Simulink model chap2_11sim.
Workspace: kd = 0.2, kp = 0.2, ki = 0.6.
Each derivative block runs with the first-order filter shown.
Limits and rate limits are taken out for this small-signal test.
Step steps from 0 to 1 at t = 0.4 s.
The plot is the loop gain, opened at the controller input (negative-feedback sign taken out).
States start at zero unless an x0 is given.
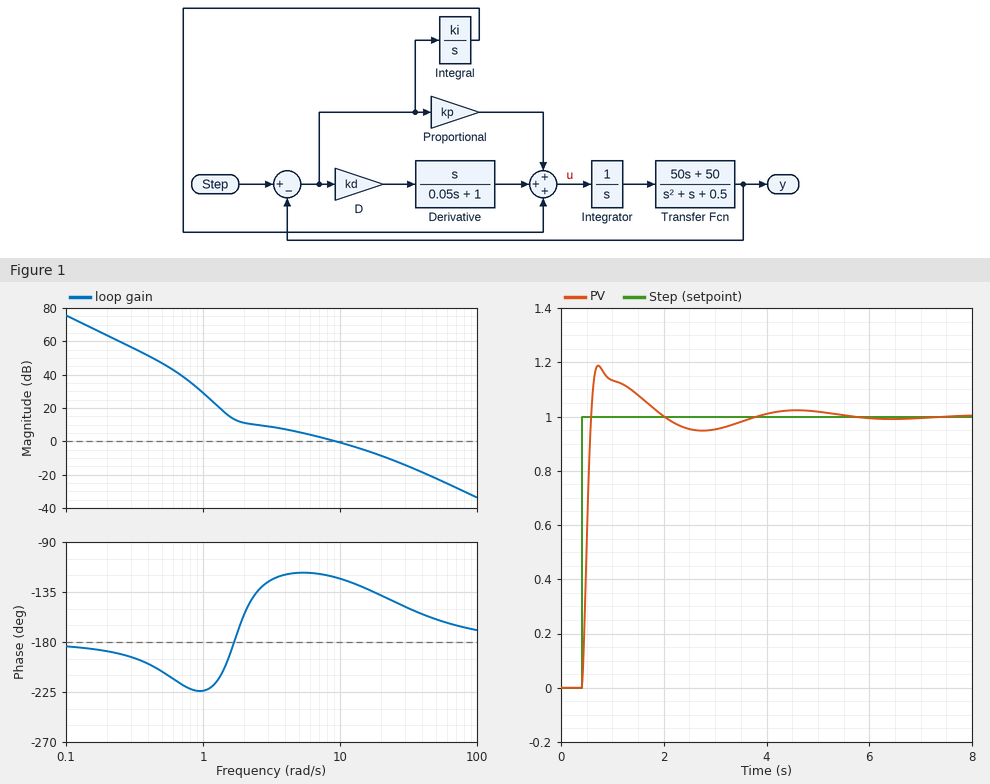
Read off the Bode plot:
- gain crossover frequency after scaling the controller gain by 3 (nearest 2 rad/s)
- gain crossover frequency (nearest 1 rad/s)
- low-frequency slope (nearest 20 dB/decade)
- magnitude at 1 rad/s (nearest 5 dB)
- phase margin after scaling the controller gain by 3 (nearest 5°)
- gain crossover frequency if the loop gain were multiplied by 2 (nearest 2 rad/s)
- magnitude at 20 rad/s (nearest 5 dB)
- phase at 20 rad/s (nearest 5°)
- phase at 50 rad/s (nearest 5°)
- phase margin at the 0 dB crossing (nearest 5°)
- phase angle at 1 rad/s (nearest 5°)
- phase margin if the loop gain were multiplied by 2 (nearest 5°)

22 rad/s
9 rad/s
-40 dB/decade
30 dB
40°
16 rad/s
-10 dB
-140°
-160°
60°
-225°
45°
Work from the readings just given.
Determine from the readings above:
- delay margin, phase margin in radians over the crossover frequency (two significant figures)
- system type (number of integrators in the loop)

0.12 s
2
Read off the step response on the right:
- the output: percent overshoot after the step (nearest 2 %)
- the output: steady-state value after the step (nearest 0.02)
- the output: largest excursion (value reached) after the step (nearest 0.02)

18 %
1.00
1.18
